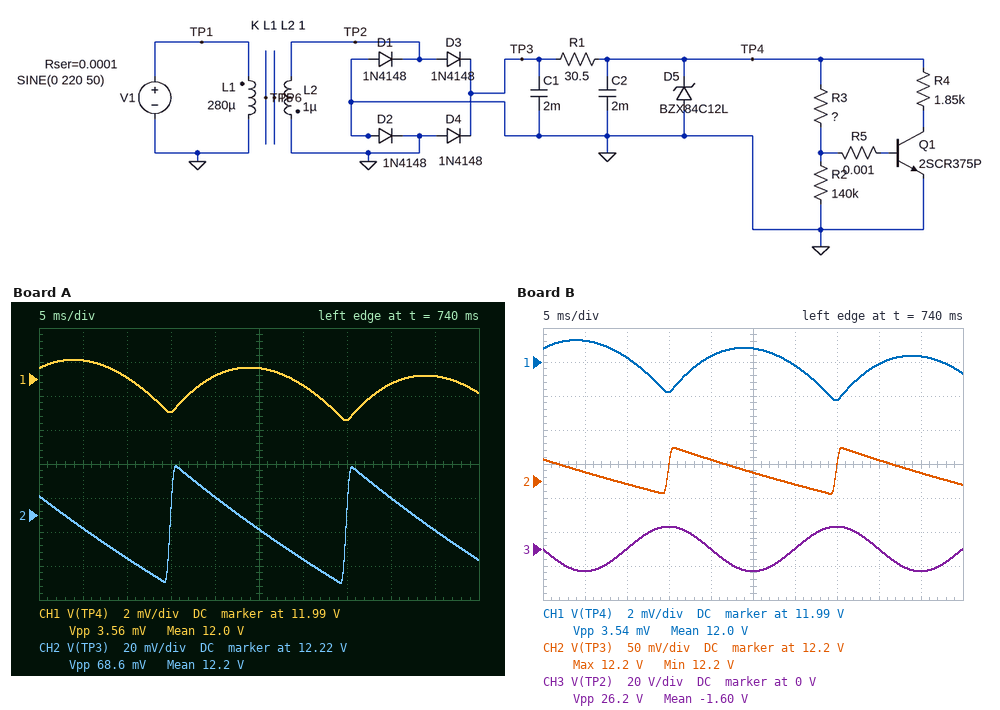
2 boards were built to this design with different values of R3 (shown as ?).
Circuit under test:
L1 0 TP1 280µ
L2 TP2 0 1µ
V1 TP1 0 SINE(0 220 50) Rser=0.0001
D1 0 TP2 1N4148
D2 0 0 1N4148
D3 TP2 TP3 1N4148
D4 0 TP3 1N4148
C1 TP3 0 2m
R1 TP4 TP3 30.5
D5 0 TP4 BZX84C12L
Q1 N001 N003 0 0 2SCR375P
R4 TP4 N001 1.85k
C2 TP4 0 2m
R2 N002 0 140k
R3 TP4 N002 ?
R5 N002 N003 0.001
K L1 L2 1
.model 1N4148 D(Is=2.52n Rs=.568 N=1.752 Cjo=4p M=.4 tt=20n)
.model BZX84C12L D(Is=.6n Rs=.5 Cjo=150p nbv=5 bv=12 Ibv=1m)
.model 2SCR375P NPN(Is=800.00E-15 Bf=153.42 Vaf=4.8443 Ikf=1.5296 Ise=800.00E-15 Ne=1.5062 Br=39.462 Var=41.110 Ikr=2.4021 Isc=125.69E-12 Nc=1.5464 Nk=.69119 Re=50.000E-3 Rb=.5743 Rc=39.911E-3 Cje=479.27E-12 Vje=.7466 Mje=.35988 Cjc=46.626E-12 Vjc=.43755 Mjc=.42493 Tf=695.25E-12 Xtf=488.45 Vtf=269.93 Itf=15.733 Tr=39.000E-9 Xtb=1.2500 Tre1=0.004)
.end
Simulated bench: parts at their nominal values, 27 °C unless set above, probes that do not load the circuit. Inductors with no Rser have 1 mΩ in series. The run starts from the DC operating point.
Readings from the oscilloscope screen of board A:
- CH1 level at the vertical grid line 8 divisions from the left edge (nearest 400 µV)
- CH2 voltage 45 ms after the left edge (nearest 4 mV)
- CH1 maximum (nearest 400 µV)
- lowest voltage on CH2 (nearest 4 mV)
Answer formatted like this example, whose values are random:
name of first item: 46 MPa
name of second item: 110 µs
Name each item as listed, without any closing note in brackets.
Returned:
CH1 level at the vertical grid line 8 divisions from the left edge: 11.9876 V
CH2 voltage 45 ms after the left edge: 12.212 V
CH1 maximum: 11.9892 V
lowest voltage on CH2: 12.180 V
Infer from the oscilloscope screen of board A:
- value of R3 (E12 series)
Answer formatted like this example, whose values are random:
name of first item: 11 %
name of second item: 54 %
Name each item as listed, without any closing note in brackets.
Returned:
value of R3: 120 kΩ
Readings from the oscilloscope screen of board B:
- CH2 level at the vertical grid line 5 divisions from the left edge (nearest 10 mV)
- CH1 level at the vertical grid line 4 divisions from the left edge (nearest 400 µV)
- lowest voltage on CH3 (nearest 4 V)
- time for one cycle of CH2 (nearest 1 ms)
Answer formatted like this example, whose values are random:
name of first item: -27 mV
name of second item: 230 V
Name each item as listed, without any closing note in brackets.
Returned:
CH2 level at the vertical grid line 5 divisions from the left edge: 12.21 V
CH1 level at the vertical grid line 4 divisions from the left edge: 11.9904 V
lowest voltage on CH3: -12 V
time for one cycle of CH2: 20 ms
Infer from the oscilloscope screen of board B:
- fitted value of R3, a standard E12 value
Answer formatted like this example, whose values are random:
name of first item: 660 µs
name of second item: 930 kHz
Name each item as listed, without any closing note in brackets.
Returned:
fitted value of R3, a standard E12 value: 180 kΩ
